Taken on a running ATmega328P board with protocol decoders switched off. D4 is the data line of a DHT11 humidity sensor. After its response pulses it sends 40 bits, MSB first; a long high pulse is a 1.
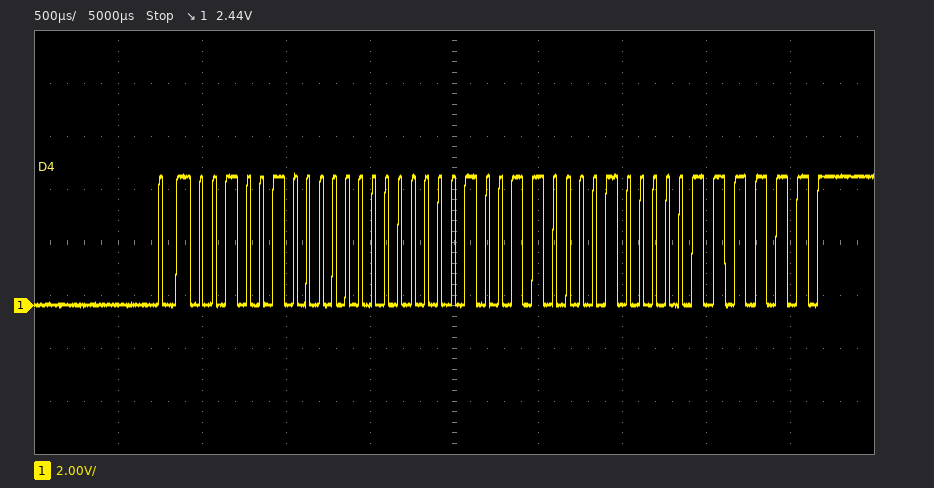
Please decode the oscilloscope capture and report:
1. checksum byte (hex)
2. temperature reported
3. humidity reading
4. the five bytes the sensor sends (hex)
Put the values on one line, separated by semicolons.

0x3F; 19.8 °C; 36 %; 24 00 13 08 3F
